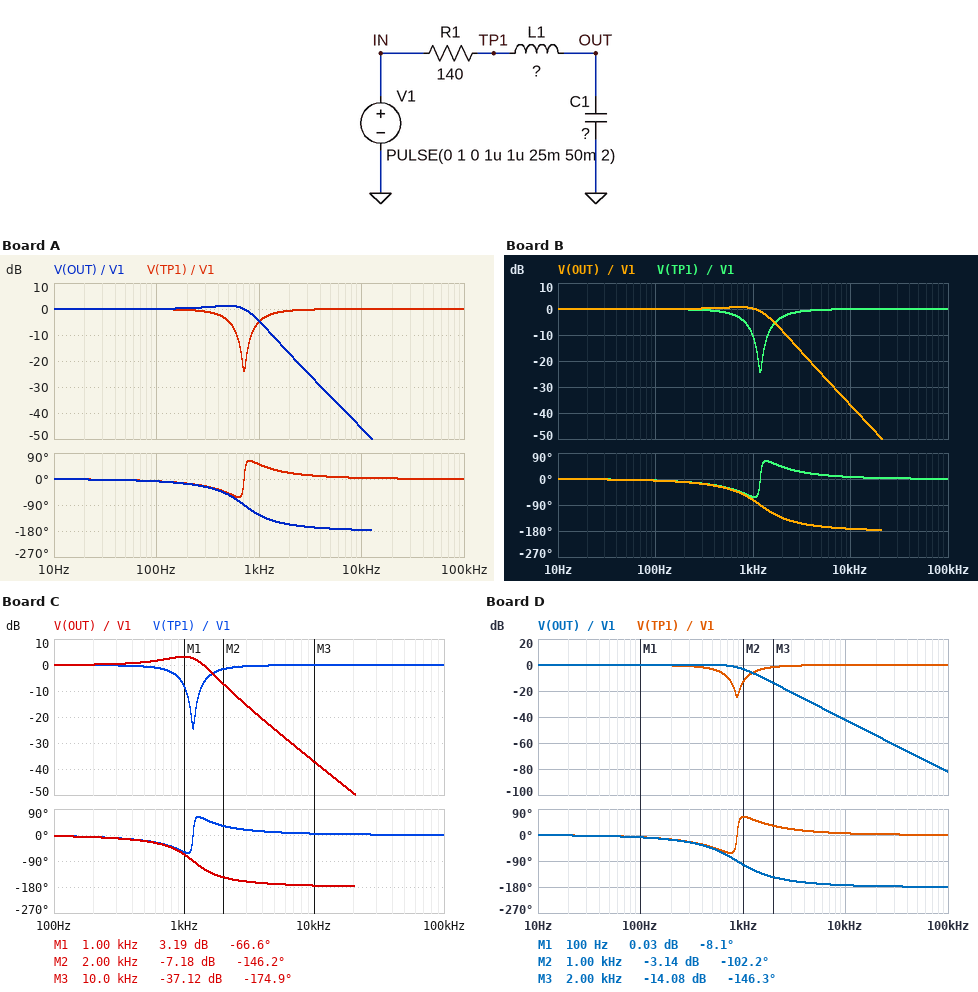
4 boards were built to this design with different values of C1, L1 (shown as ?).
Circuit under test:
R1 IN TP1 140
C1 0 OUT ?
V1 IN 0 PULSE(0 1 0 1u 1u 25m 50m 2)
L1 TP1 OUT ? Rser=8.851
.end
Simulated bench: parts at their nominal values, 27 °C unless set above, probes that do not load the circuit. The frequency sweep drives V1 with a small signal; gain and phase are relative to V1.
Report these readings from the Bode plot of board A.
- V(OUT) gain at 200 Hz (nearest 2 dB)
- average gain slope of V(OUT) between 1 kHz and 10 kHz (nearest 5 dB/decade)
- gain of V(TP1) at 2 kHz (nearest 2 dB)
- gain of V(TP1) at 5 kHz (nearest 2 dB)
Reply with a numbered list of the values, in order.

1. 0 dB
2. -40 dB/decade
3. 0 dB
4. 0 dB
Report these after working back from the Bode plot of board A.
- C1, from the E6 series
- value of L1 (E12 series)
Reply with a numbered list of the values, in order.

1. 1.5 µF
2. 33 mH
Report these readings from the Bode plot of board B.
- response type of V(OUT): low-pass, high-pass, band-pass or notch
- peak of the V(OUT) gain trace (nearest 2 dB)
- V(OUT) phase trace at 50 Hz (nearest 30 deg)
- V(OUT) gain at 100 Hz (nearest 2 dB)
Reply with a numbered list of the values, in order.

1. low-pass
2. 0 dB
3. 0 deg
4. 0 dB
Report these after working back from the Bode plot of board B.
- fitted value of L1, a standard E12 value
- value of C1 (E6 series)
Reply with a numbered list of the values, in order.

1. 18 mH
2. 1 µF
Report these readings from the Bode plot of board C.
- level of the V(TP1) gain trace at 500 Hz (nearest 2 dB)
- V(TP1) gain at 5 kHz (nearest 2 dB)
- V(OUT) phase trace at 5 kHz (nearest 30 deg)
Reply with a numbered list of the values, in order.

1. 0 dB
2. 0 dB
3. -180 deg
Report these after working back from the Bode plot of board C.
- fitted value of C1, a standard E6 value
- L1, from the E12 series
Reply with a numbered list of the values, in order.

1. 680 nF
2. 27 mH
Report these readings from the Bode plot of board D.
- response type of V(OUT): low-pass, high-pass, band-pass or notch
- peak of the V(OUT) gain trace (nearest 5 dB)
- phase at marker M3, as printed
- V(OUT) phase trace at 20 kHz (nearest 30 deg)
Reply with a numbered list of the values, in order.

1. low-pass
2. 0 dB
3. -146.3 deg
4. -180 deg
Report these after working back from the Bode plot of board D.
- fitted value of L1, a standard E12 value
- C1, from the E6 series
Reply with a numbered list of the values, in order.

1. 22 mH
2. 1.5 µF
